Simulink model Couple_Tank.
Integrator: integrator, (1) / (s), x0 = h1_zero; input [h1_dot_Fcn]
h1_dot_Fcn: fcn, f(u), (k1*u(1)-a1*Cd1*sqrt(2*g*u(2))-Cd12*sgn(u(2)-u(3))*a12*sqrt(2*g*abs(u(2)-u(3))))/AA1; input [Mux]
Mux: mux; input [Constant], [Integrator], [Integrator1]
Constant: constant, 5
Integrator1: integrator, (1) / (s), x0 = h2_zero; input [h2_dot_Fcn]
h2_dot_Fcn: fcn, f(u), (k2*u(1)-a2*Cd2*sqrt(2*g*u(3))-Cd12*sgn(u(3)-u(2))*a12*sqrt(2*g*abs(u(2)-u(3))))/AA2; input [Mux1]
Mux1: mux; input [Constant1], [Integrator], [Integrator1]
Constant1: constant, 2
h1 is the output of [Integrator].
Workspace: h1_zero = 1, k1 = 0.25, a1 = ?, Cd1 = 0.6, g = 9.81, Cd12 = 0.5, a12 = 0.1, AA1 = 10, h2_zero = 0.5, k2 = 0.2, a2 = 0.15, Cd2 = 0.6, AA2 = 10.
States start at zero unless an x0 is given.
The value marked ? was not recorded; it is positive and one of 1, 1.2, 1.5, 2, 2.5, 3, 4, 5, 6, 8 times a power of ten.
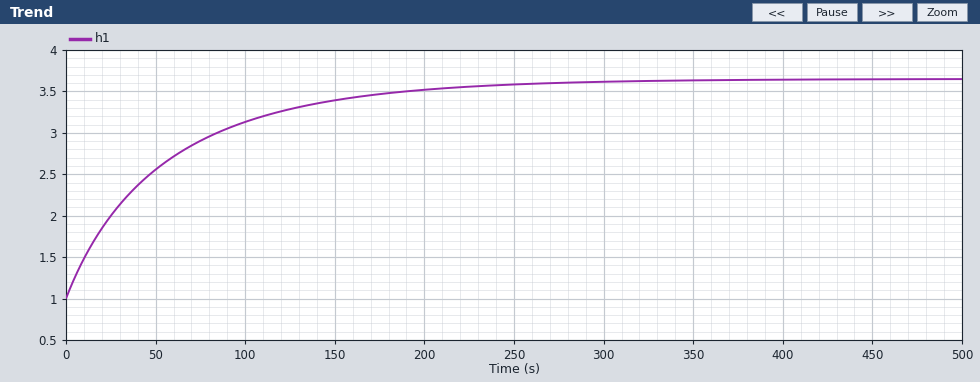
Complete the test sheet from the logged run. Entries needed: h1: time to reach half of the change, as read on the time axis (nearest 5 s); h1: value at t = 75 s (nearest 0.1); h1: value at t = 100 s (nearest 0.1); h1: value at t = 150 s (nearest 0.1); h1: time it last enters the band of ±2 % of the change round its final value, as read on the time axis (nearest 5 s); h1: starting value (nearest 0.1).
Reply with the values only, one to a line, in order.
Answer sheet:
40 s
2.9
3.1
3.4
270 s
1.0
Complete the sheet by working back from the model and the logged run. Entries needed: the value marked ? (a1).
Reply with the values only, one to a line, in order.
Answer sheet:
0.2
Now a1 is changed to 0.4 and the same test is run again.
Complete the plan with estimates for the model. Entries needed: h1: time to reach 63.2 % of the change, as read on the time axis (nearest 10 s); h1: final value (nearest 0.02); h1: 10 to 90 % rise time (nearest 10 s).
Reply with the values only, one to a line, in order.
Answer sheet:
50 s
1.28
80 s
